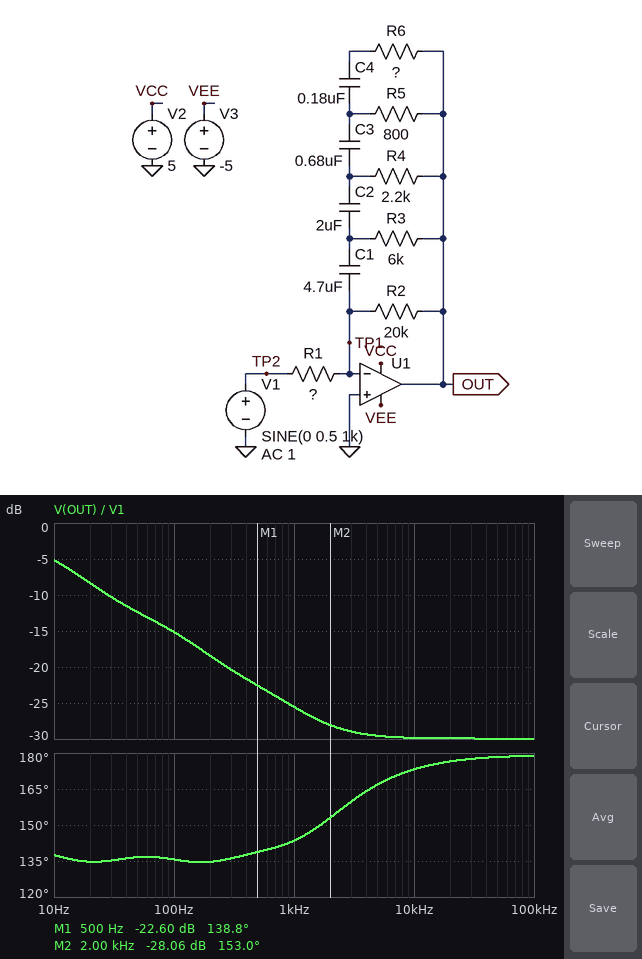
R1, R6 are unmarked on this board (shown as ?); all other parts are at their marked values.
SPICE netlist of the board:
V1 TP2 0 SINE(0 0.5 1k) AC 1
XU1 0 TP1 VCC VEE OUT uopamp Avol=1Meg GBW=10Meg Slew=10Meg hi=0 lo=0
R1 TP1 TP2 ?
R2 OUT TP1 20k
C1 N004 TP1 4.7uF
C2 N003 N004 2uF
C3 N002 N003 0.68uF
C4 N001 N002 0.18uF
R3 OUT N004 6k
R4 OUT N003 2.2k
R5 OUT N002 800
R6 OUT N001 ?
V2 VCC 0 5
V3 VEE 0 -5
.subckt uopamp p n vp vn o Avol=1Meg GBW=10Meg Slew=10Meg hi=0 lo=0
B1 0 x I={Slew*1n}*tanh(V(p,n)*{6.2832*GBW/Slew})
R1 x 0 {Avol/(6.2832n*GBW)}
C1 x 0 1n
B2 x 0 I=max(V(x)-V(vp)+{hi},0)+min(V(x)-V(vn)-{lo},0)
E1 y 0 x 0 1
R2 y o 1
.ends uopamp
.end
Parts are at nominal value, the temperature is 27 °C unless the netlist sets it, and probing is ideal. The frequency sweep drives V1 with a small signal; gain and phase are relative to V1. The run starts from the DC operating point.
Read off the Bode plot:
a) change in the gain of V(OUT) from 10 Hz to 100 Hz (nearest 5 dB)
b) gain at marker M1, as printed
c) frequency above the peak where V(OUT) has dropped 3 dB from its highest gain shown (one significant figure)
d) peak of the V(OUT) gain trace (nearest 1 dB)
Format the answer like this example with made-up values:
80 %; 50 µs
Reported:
-10 dB; -22.60 dB; 20 Hz; -5 dB
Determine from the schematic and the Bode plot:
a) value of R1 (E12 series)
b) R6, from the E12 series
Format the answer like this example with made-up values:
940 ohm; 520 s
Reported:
10 kΩ; 820 Ω
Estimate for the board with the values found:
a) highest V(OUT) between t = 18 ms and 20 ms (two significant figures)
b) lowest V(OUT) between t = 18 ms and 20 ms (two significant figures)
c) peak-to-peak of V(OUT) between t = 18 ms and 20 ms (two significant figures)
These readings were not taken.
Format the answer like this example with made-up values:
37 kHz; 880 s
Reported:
25 mV; -28 mV; 53 mV
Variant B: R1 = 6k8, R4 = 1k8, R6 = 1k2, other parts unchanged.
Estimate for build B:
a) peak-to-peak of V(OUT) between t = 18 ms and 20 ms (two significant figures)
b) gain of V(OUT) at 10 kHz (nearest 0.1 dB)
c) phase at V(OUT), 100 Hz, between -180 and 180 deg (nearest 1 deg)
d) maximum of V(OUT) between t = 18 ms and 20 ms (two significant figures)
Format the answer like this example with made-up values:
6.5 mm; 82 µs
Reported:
73 mV; -25.7 dB; 135 deg; 35 mV
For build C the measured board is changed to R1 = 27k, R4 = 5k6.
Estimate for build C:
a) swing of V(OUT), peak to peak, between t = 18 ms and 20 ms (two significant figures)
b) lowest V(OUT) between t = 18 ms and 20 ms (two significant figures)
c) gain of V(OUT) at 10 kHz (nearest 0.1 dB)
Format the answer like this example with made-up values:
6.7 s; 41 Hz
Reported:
22 mV; -11 mV; -37.7 dB
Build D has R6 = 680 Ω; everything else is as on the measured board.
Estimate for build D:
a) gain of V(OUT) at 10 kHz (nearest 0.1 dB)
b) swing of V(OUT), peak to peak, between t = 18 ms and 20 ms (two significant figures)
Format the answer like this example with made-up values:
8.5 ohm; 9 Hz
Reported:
-30.5 dB; 54 mV
